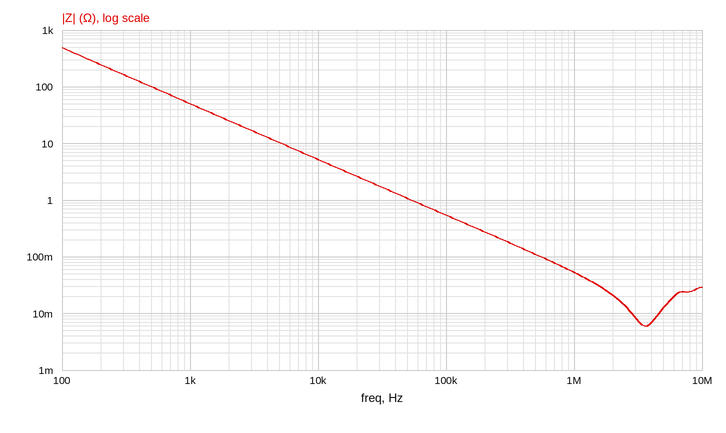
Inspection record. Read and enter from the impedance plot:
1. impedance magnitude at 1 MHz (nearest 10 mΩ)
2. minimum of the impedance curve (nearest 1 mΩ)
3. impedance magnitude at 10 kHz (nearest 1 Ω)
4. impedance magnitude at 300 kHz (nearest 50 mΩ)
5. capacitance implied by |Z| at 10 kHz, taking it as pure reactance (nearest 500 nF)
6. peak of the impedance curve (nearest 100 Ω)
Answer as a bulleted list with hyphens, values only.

- 50 mΩ
- 6 mΩ
- 5 Ω
- 200 mΩ
- 3.0 µF
- 500 Ω
